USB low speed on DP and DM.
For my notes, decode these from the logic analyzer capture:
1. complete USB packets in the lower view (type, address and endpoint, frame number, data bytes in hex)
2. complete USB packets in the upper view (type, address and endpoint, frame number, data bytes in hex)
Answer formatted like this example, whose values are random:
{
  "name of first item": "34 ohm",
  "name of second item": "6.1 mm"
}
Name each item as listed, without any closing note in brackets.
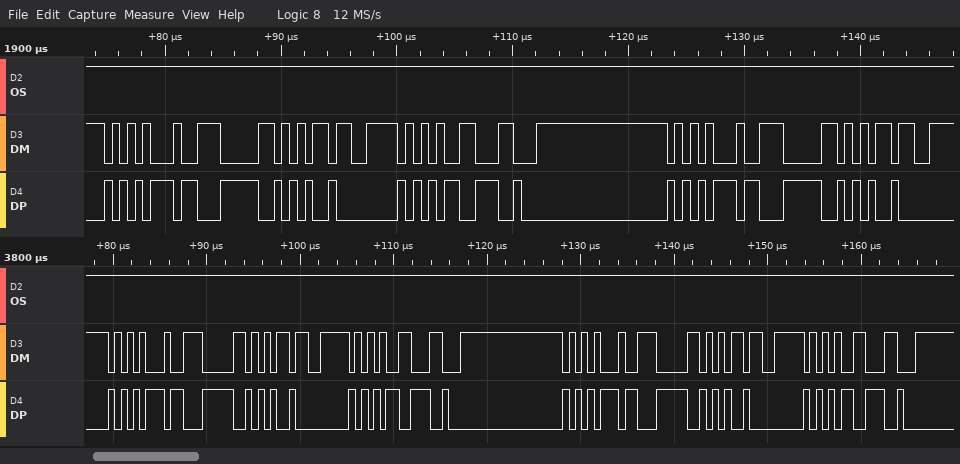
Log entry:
{
  "complete USB packets in the lower view": "IN ADDR 47 EP 0, NAK, IN ADDR 47 EP 0, NAK",
  "complete USB packets in the upper view": "IN ADDR 47 EP 0, NAK, IN ADDR 47 EP 0"
}
